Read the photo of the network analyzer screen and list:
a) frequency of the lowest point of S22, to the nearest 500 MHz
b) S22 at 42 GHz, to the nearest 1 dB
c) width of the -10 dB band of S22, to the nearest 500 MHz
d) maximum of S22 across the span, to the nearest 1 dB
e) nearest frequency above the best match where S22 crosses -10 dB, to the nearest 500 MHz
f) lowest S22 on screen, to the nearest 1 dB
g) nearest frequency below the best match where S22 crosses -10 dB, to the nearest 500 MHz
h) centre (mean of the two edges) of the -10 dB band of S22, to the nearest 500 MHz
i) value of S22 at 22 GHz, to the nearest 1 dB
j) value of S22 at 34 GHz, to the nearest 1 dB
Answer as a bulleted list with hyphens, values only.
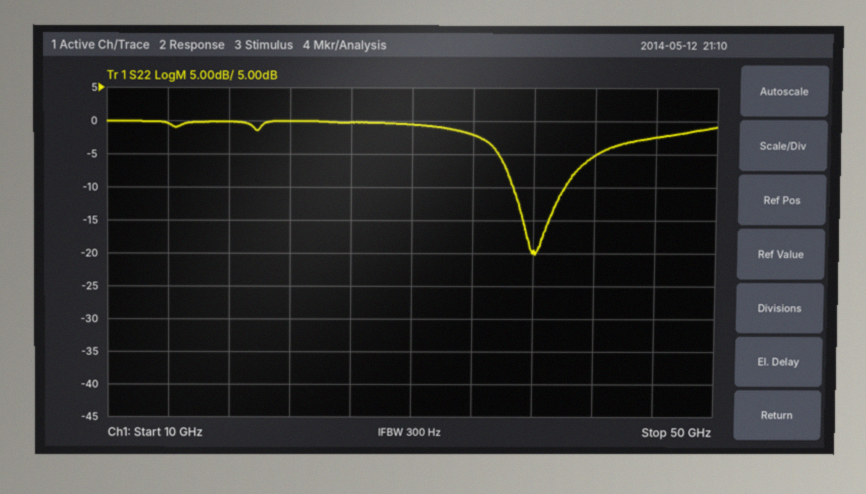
- 38.0 GHz
- -5 dB
- 3.5 GHz
- 0 dB
- 40.0 GHz
- -20 dB
- 36.5 GHz
- 38.5 GHz
- 0 dB
- -2 dB
